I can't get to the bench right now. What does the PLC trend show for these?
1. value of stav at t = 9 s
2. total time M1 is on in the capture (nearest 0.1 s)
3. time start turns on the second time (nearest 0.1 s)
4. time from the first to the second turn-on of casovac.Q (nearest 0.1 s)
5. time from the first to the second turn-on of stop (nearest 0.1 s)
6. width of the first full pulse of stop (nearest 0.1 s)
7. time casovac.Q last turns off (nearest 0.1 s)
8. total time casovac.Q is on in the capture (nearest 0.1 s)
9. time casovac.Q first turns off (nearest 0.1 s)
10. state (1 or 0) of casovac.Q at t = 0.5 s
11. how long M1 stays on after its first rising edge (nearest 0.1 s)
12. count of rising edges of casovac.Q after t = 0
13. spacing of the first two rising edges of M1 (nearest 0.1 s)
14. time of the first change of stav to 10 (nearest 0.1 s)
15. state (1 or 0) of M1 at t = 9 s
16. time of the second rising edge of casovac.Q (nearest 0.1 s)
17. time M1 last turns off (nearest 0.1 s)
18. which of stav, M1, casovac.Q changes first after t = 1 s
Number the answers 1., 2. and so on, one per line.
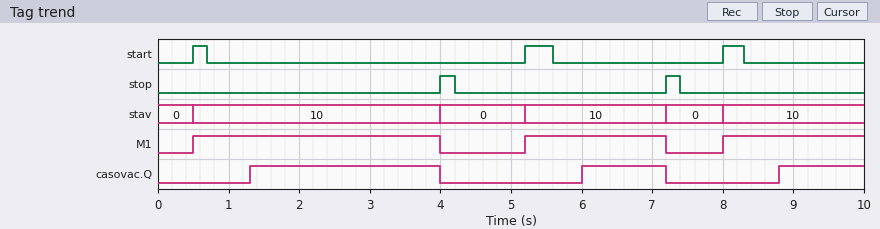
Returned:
1. 10
2. 7.5 s
3. 5.2 s
4. 4.7 s
5. 3.2 s
6. 0.2 s
7. 7.2 s
8. 5.1 s
9. 4.0 s
10. 0
11. 3.5 s
12. 3
13. 4.7 s
14. 0.5 s
15. 1
16. 6.0 s
17. 7.2 s
18. casovac.Q
